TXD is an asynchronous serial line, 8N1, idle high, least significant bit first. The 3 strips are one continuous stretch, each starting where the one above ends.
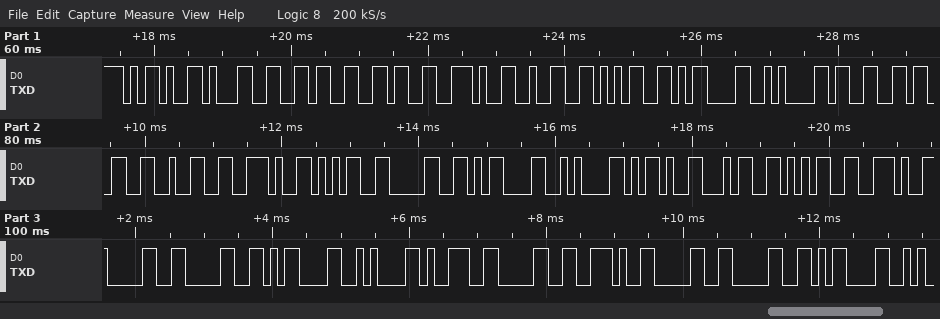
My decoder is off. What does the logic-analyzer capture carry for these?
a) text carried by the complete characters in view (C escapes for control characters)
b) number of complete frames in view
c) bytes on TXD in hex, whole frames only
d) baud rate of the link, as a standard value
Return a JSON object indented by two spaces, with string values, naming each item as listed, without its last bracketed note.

{
  "text carried by the complete characters in view": "\"-166.25\\r\\n332.50\\r\\n-45.00\\r\\n90.00\\r\"",
  "number of complete frames in view": "31",
  "bytes on TXD in hex, whole frames only": "2D 31 36 36 2E 32 35 0D 0A 33 33 32 2E 35 30 0D 0A 2D 34 35 2E 30 30 0D 0A 39 30 2E 30 30 0D",
  "baud rate of the link, as a standard value": "9600 baud"
}
